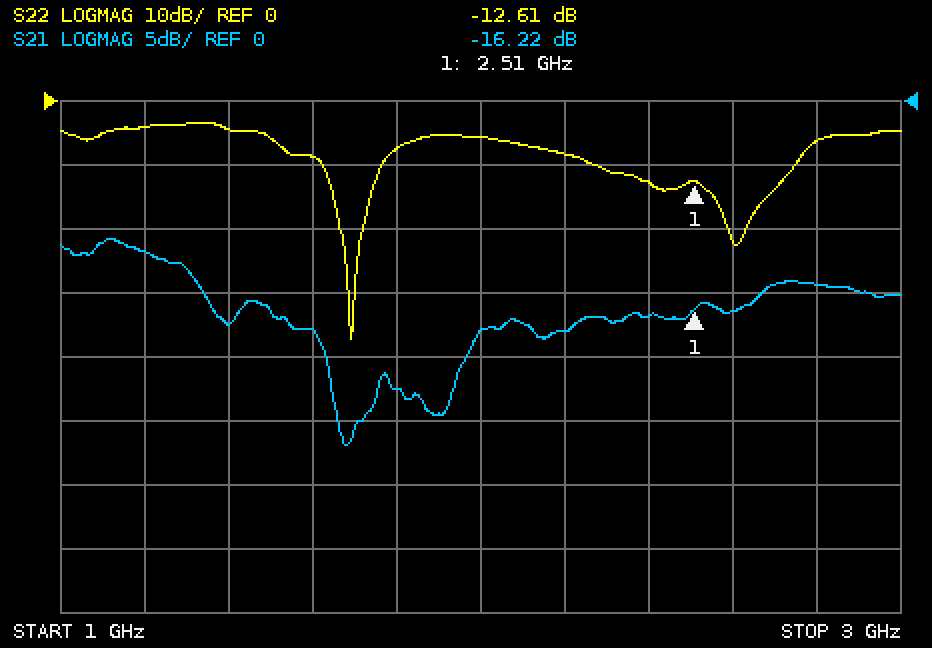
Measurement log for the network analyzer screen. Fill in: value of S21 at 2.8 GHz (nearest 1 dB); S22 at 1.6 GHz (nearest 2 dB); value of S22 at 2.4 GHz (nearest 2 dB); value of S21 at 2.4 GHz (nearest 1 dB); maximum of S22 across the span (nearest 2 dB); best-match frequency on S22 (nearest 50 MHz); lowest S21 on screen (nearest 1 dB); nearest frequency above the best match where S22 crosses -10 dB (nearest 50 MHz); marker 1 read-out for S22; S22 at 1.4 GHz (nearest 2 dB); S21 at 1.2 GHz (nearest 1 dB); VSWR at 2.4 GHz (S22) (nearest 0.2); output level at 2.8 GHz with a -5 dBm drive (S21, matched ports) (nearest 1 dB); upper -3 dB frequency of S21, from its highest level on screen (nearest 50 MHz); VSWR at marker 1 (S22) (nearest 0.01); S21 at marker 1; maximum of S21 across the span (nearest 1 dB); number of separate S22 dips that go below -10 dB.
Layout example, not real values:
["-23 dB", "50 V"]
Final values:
["-14 dB", "-8 dB", "-12 dB", "-17 dB", "-4 dB", "1.70 GHz", "-27 dB", "1.75 GHz", "-12.61 dB", "-4 dB", "-12 dB", "1.6", "-19 dBm", "1.30 GHz", "1.61", "-16.22 dB", "-11 dB", "2"]
